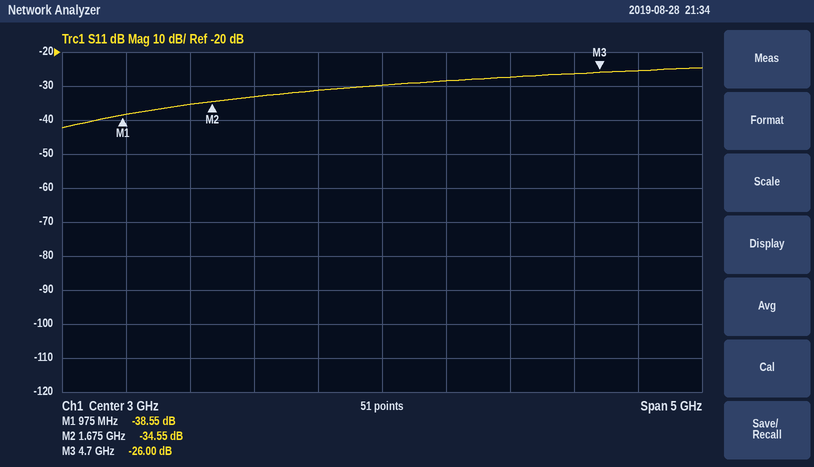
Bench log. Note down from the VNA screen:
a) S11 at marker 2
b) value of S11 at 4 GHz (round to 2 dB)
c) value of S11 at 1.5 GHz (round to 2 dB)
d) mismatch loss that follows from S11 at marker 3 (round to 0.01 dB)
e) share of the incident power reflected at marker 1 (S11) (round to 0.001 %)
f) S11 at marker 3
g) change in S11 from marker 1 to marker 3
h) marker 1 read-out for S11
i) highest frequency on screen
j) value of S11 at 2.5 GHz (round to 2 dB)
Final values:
-34.55 dB
-28 dB
-36 dB
0.01 dB
0.014 %
-26.00 dB
12.55 dB
-38.55 dB
5.5 GHz
-32 dB
